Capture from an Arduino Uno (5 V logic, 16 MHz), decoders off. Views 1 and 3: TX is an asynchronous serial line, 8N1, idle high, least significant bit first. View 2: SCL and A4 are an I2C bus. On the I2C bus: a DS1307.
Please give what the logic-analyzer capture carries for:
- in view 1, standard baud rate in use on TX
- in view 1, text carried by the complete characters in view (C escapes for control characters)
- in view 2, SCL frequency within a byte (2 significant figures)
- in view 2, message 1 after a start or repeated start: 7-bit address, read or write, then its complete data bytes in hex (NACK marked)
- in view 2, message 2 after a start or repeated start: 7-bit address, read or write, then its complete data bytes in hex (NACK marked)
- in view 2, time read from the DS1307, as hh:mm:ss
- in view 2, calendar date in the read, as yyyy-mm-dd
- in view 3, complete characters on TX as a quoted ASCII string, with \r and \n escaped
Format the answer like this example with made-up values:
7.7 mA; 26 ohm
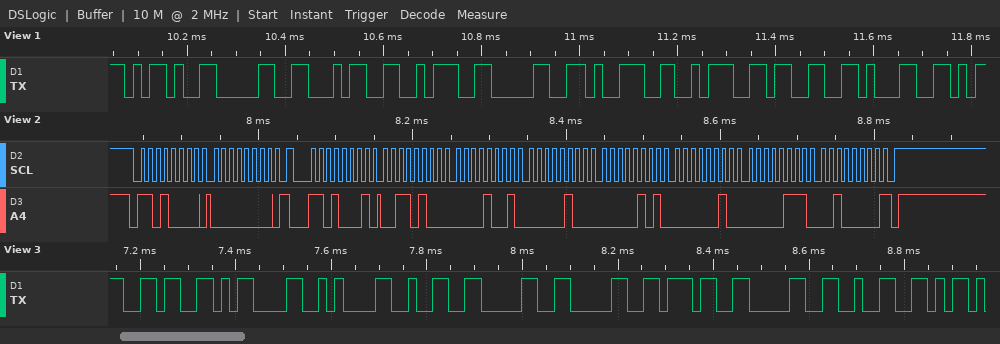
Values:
57600 baud; "-04:09:31"; 100 kHz; 0x68 write: 00; 0x68 read: 34 09 04 05 02 07 20 NACK; 04:09:34; 2020-07-02; "6\r\n200702"
